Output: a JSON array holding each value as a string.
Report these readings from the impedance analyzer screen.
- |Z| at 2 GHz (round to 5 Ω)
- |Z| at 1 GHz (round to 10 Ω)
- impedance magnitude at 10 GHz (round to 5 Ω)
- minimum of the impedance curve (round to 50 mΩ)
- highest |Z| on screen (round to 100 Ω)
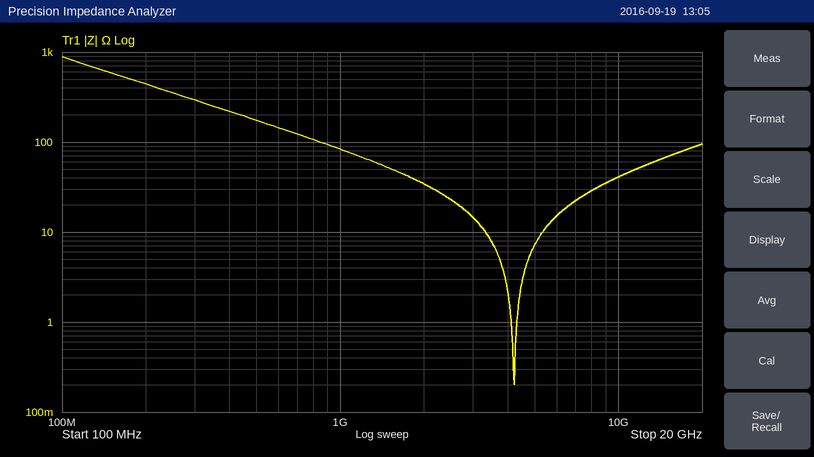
["35 Ω", "80 Ω", "40 Ω", "200 mΩ", "900 Ω"]
